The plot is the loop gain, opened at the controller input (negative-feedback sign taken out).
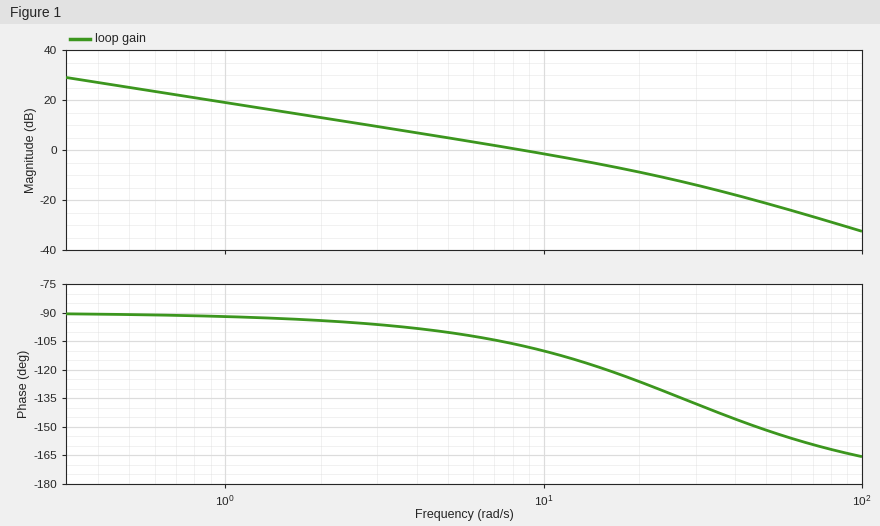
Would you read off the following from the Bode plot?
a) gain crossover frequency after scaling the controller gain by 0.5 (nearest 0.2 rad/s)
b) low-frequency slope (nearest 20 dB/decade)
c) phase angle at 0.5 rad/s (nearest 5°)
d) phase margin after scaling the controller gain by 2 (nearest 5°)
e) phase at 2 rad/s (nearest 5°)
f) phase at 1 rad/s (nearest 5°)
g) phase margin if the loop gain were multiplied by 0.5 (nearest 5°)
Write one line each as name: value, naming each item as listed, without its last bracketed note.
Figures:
gain crossover frequency after scaling the controller gain by 0.5: 4.4 rad/s
low-frequency slope: -20 dB/decade
phase angle at 0.5 rad/s: -90°
phase margin after scaling the controller gain by 2: 60°
phase at 2 rad/s: -95°
phase at 1 rad/s: -90°
phase margin if the loop gain were multiplied by 0.5: 80°
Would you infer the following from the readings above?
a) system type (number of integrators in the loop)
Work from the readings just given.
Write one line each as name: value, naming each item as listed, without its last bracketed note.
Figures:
system type: 1
